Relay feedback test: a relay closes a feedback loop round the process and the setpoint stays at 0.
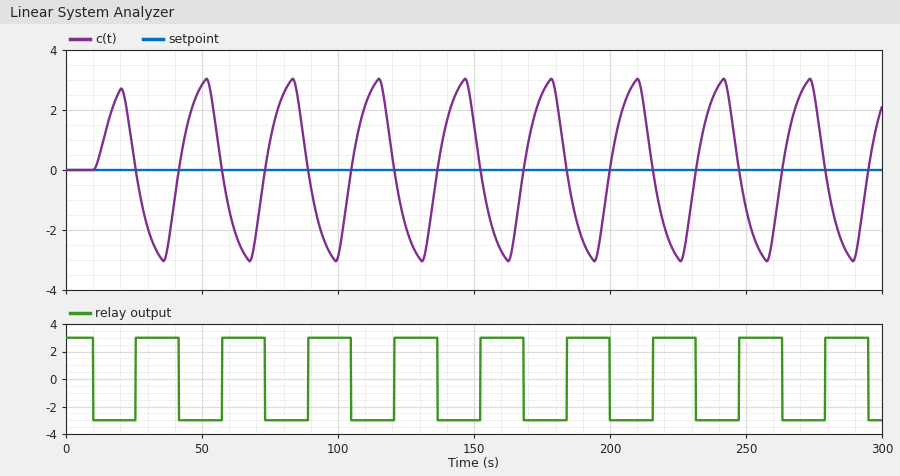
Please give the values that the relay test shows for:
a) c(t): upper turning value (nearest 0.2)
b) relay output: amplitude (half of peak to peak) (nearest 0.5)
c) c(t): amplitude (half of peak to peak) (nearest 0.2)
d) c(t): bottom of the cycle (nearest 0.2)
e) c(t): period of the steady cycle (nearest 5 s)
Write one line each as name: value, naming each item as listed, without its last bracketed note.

c(t): upper turning value: 3.0
relay output: amplitude (half of peak to peak): 3.0
c(t): amplitude (half of peak to peak): 3.0
c(t): bottom of the cycle: -3.0
c(t): period of the steady cycle: 30 s
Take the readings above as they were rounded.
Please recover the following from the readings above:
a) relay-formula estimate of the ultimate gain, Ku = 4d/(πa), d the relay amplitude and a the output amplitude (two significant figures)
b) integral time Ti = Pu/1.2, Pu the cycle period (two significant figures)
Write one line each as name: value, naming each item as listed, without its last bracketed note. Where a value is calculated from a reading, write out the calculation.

relay-formula estimate of the ultimate gain, Ku = 4d/(πa), d the relay amplitude and a the output amplitude: 4 × 3 / (π × 3) = 1.3
integral time Ti = Pu/1.2, Pu the cycle period: 30 / 1.2 = 25 s
